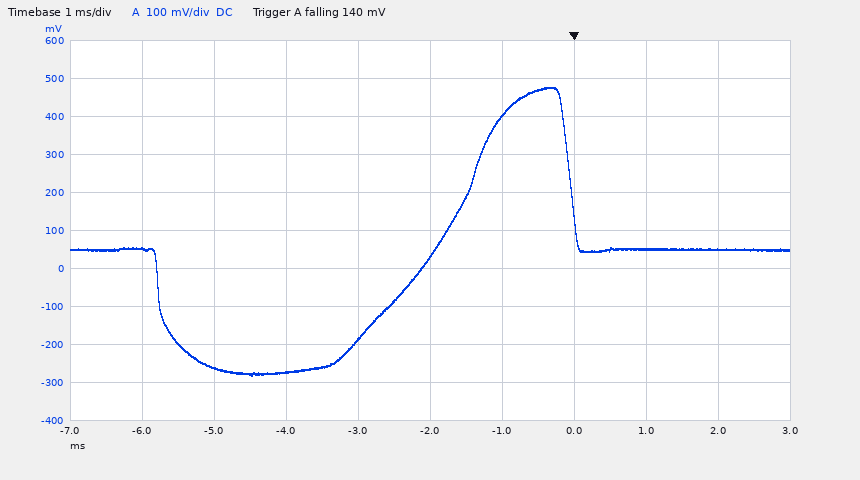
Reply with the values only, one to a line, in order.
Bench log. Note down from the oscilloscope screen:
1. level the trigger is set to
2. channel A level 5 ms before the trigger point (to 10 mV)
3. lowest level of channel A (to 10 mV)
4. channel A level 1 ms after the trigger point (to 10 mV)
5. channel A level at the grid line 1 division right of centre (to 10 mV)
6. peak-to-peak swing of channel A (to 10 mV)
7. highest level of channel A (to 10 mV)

140 mV
-260 mV
-280 mV
50 mV
400 mV
760 mV
480 mV
